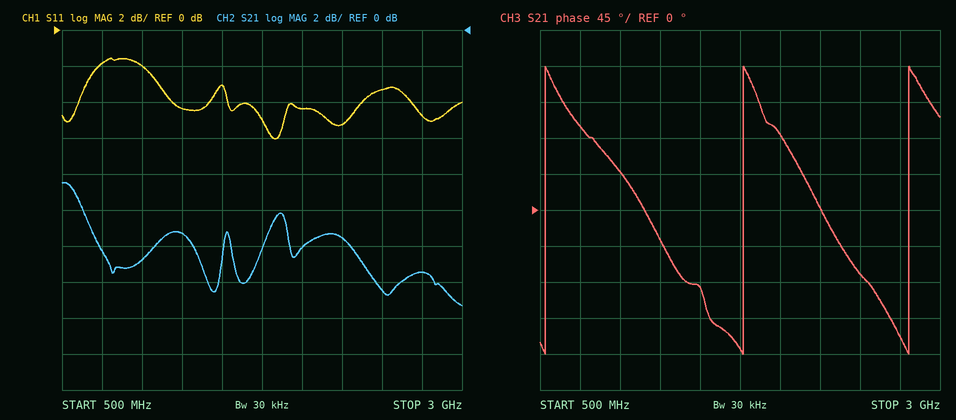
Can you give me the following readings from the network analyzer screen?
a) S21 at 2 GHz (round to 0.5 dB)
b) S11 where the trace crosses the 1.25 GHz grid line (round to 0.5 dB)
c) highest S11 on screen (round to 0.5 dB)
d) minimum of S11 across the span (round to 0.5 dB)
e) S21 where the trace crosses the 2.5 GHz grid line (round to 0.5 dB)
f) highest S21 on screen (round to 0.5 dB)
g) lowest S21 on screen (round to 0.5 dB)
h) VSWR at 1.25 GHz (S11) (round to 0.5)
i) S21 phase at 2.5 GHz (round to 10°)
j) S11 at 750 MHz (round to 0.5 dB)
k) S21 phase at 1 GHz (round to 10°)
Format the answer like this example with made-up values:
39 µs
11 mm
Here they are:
-12.0 dB
-4.5 dB
-1.5 dB
-6.0 dB
-14.5 dB
-8.5 dB
-15.5 dB
4.0
-80°
-2.0 dB
50°
